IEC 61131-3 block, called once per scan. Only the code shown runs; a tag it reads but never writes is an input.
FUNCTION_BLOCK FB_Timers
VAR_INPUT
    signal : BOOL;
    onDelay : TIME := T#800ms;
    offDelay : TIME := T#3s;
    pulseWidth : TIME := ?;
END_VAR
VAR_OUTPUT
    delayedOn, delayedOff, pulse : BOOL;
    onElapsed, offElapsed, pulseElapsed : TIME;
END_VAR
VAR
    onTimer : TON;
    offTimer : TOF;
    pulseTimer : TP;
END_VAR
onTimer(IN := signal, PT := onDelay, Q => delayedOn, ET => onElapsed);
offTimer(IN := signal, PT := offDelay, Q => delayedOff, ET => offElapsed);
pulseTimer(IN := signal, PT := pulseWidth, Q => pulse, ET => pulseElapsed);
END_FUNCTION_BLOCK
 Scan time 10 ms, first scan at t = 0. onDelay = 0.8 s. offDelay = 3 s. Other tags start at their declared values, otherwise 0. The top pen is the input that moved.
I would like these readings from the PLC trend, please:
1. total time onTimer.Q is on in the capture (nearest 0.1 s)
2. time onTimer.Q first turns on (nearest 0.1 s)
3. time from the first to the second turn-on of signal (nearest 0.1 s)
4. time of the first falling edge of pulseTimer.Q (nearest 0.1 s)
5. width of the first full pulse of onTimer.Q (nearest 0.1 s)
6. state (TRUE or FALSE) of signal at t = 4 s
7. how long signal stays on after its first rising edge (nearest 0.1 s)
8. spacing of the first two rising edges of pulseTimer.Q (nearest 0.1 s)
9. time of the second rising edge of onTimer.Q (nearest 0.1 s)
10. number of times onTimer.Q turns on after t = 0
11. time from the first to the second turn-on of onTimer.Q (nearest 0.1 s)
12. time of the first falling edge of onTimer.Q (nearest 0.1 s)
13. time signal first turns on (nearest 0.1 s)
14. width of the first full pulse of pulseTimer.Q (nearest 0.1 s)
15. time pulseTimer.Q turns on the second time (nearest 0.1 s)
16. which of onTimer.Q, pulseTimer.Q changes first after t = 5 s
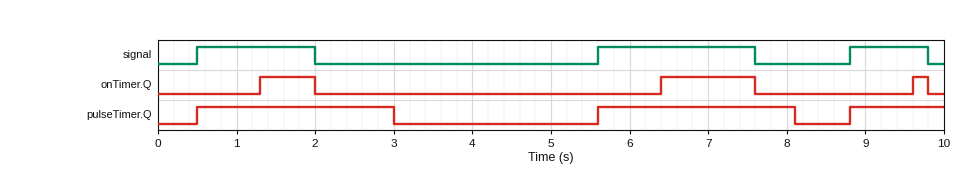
2.1 s
1.3 s
5.1 s
3.0 s
0.7 s
FALSE
1.5 s
5.1 s
6.4 s
3
5.1 s
2.0 s
0.5 s
2.5 s
5.6 s
pulseTimer.Q
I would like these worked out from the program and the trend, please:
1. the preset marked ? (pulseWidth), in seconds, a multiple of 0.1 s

2.5 s
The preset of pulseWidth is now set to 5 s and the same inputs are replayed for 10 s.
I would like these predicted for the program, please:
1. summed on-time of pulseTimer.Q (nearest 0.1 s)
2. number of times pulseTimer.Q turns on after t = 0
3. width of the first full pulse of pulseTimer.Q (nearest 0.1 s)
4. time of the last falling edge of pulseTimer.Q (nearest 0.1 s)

9.4 s
2
5.0 s
5.5 s
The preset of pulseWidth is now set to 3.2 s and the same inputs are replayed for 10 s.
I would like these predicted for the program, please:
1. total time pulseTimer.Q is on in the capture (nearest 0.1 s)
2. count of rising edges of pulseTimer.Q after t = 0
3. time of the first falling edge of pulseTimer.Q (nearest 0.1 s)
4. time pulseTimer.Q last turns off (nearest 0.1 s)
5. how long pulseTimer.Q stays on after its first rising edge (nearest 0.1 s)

6.4 s
2
3.7 s
8.8 s
3.2 s
